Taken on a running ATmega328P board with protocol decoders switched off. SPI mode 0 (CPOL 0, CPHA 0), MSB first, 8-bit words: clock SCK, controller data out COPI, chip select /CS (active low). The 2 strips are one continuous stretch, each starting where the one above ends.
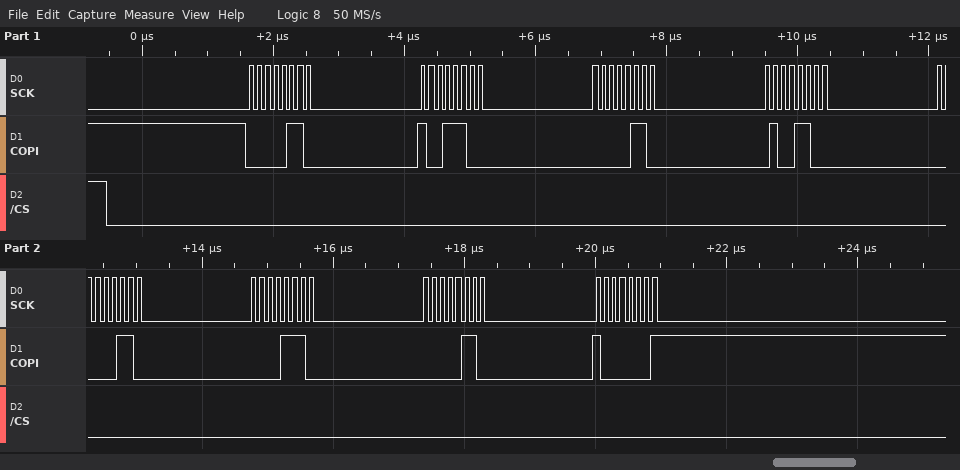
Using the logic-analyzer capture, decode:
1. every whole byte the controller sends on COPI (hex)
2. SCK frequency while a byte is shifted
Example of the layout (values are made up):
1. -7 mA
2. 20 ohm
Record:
1. 06 9C 06 4C 06 0E 06 81
2. 8 MHz
